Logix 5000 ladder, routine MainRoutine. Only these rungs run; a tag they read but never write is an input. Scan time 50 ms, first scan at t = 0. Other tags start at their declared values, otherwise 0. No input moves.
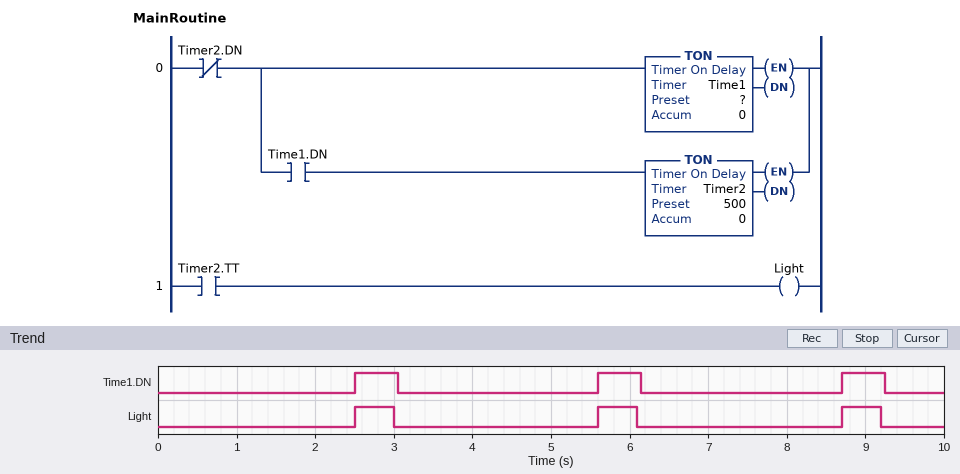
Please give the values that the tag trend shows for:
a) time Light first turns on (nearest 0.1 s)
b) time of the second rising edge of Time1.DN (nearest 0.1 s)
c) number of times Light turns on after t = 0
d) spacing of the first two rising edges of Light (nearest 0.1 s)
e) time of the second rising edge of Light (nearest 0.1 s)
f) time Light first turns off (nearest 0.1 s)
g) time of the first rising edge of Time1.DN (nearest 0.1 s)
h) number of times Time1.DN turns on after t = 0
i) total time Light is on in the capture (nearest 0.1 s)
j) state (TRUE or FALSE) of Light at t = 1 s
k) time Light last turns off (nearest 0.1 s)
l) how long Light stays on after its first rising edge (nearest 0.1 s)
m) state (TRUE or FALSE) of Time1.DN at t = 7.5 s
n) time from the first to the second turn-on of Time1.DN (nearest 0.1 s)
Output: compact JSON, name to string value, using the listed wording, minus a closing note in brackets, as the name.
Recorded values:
{"time Light first turns on": "2.5 s", "time of the second rising edge of Time1.DN": "5.6 s", "number of times Light turns on after t = 0": "3", "spacing of the first two rising edges of Light": "3.1 s", "time of the second rising edge of Light": "5.6 s", "time Light first turns off": "3.0 s", "time of the first rising edge of Time1.DN": "2.5 s", "number of times Time1.DN turns on after t = 0": "3", "total time Light is on in the capture": "1.5 s", "state (TRUE or FALSE) of Light at t = 1 s": "FALSE", "time Light last turns off": "9.2 s", "how long Light stays on after its first rising edge": "0.5 s", "state (TRUE or FALSE) of Time1.DN at t = 7.5 s": "FALSE", "time from the first to the second turn-on of Time1.DN": "3.1 s"}
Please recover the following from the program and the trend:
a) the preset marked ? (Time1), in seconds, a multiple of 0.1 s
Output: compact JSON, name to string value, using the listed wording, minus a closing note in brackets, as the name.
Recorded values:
{"the preset marked ? (Time1), in seconds, a multiple of 0.1 s": "2.5 s"}
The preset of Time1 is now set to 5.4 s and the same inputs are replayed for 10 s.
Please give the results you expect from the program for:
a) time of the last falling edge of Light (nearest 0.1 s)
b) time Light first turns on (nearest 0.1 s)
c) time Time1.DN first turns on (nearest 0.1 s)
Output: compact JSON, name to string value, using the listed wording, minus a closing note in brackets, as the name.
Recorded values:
{"time of the last falling edge of Light": "5.9 s", "time Light first turns on": "5.4 s", "time Time1.DN first turns on": "5.4 s"}
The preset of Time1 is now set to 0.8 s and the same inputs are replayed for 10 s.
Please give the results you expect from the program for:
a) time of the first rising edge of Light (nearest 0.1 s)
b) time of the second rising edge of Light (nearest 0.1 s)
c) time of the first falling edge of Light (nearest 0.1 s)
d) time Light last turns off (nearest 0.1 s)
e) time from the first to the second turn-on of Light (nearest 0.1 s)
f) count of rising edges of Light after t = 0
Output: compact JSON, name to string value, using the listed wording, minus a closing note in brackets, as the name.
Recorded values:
{"time of the first rising edge of Light": "0.8 s", "time of the second rising edge of Light": "2.2 s", "time of the first falling edge of Light": "1.3 s", "time Light last turns off": "9.7 s", "time from the first to the second turn-on of Light": "1.4 s", "count of rising edges of Light after t = 0": "7"}
